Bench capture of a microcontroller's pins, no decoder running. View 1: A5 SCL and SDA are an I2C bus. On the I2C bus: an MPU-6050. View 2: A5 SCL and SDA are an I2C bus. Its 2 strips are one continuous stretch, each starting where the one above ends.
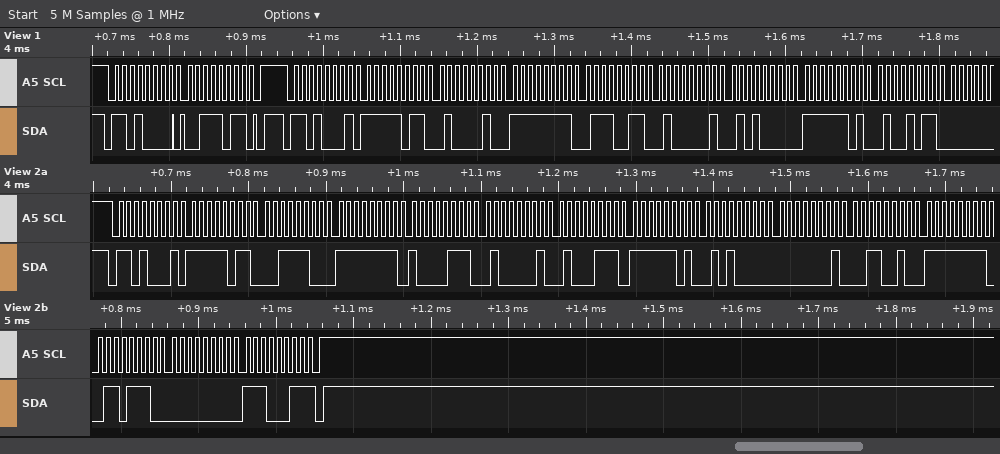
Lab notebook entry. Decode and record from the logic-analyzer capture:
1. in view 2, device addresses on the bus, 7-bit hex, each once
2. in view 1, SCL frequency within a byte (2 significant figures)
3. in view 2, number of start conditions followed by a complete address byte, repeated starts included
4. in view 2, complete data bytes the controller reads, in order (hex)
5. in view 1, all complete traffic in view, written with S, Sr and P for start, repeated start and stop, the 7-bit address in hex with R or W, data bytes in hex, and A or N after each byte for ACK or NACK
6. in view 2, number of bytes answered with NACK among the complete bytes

0x68
100 kHz
1
FB 3C FF 87 41 47 FD 50 01 32 FF 6E 00 E3
S 68W A 3B A P S 68R A FB A 42 A FF A 73 A 41 A 50 A FD A 4B A
1
